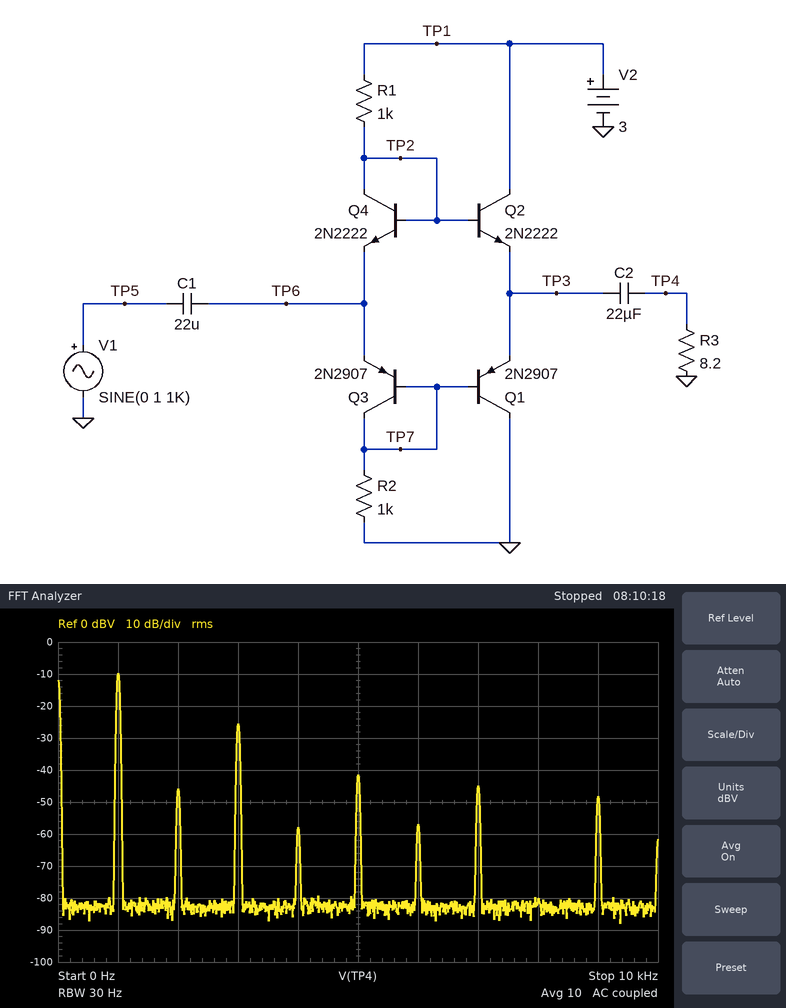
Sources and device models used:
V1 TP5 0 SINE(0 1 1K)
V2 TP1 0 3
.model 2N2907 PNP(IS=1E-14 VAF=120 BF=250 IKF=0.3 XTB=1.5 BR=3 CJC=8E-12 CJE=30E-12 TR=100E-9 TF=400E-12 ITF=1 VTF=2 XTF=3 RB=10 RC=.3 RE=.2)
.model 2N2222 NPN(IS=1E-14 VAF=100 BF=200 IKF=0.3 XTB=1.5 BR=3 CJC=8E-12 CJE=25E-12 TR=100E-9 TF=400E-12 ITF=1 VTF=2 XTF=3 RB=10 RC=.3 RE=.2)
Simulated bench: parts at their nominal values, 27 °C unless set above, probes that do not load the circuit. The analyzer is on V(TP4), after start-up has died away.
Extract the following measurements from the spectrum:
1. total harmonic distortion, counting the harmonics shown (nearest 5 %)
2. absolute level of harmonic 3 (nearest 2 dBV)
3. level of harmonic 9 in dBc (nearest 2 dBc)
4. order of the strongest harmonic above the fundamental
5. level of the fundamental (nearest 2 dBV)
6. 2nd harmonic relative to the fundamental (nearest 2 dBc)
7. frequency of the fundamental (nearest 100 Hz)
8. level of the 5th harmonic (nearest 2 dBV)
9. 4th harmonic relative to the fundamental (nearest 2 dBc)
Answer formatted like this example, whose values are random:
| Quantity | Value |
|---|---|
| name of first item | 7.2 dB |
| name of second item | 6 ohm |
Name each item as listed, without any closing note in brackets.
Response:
| Quantity | Value |
|---|---|
| total harmonic distortion, counting the harmonics shown | 15 % |
| absolute level of harmonic 3 | -26 dBV |
| level of harmonic 9 in dBc | -38 dBc |
| order of the strongest harmonic above the fundamental | 3 |
| level of the fundamental | -10 dBV |
| 2nd harmonic relative to the fundamental | -36 dBc |
| frequency of the fundamental | 1.0 kHz |
| level of the 5th harmonic | -42 dBV |
| 4th harmonic relative to the fundamental | -48 dBc |
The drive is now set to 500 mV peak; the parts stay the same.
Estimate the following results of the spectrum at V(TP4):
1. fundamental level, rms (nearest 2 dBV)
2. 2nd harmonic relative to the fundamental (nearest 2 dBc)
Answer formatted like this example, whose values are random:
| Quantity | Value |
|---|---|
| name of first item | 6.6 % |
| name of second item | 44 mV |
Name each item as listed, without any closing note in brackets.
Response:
| Quantity | Value |
|---|---|
| fundamental level, rms | -14 dBV |
| 2nd harmonic relative to the fundamental | -54 dBc |
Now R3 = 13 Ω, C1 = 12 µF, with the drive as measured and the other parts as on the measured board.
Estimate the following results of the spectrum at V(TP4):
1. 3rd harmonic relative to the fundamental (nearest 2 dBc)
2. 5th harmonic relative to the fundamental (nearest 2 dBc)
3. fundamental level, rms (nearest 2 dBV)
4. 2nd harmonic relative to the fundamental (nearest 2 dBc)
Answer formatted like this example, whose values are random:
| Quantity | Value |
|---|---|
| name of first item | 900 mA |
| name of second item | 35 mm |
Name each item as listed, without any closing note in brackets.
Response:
| Quantity | Value |
|---|---|
| 3rd harmonic relative to the fundamental | -18 dBc |
| 5th harmonic relative to the fundamental | -30 dBc |
| fundamental level, rms | -8 dBV |
| 2nd harmonic relative to the fundamental | -38 dBc |
